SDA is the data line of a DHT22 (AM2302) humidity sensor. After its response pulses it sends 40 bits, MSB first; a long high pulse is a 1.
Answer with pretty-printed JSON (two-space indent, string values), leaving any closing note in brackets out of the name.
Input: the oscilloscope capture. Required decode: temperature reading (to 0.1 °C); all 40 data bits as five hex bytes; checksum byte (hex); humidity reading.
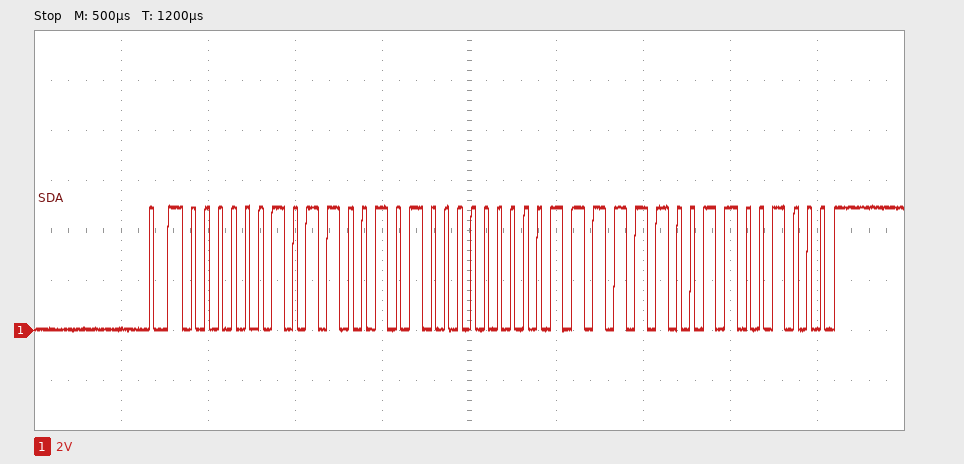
{
  "temperature reading": "25.2 °C",
  "all 40 data bits as five hex bytes": "02 CA 00 FC C8",
  "checksum byte": "0xC8",
  "humidity reading": "71.4 %"
}
